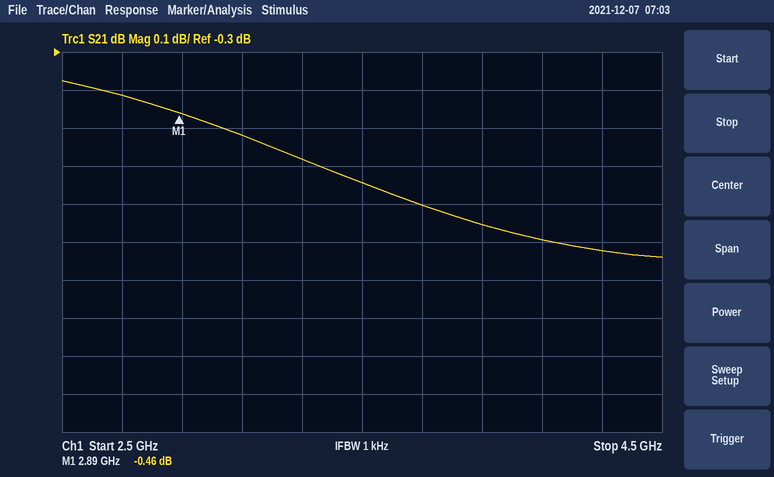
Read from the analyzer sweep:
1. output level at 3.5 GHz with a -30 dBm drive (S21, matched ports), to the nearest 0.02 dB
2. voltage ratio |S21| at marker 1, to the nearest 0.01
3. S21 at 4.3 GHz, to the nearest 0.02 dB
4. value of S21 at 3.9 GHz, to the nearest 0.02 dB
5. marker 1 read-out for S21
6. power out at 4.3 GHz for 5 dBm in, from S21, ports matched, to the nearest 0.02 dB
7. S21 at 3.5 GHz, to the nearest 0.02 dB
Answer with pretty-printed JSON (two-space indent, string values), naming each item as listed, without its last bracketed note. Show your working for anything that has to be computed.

{
  "output level at 3.5 GHz with a -30 dBm drive (S21, matched ports), to the nearest 0.02 dB": "-30 dBm + (-0.64 dB) = -30.64 dBm",
  "voltage ratio |S21| at marker 1, to the nearest 0.01": "10^(-0.46/20) ≈ 0.95",
  "S21 at 4.3 GHz, to the nearest 0.02 dB": "-0.82 dB",
  "value of S21 at 3.9 GHz, to the nearest 0.02 dB": "-0.76 dB",
  "marker 1 read-out for S21": "-0.46 dB",
  "power out at 4.3 GHz for 5 dBm in, from S21, ports matched, to the nearest 0.02 dB": "5 dBm + (-0.82 dB) = 4.18 dBm",
  "S21 at 3.5 GHz, to the nearest 0.02 dB": "-0.64 dB"
}
